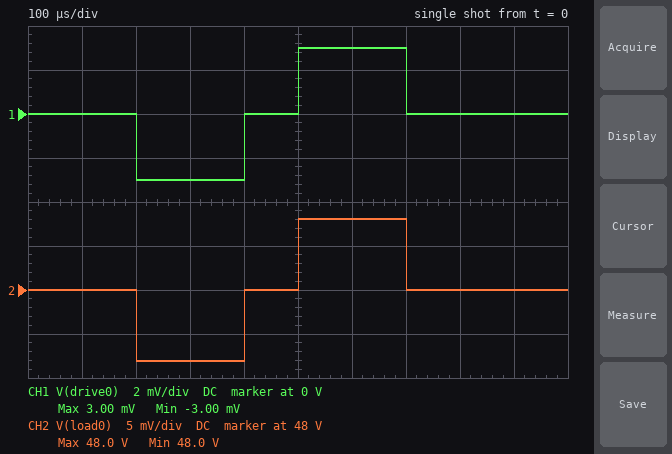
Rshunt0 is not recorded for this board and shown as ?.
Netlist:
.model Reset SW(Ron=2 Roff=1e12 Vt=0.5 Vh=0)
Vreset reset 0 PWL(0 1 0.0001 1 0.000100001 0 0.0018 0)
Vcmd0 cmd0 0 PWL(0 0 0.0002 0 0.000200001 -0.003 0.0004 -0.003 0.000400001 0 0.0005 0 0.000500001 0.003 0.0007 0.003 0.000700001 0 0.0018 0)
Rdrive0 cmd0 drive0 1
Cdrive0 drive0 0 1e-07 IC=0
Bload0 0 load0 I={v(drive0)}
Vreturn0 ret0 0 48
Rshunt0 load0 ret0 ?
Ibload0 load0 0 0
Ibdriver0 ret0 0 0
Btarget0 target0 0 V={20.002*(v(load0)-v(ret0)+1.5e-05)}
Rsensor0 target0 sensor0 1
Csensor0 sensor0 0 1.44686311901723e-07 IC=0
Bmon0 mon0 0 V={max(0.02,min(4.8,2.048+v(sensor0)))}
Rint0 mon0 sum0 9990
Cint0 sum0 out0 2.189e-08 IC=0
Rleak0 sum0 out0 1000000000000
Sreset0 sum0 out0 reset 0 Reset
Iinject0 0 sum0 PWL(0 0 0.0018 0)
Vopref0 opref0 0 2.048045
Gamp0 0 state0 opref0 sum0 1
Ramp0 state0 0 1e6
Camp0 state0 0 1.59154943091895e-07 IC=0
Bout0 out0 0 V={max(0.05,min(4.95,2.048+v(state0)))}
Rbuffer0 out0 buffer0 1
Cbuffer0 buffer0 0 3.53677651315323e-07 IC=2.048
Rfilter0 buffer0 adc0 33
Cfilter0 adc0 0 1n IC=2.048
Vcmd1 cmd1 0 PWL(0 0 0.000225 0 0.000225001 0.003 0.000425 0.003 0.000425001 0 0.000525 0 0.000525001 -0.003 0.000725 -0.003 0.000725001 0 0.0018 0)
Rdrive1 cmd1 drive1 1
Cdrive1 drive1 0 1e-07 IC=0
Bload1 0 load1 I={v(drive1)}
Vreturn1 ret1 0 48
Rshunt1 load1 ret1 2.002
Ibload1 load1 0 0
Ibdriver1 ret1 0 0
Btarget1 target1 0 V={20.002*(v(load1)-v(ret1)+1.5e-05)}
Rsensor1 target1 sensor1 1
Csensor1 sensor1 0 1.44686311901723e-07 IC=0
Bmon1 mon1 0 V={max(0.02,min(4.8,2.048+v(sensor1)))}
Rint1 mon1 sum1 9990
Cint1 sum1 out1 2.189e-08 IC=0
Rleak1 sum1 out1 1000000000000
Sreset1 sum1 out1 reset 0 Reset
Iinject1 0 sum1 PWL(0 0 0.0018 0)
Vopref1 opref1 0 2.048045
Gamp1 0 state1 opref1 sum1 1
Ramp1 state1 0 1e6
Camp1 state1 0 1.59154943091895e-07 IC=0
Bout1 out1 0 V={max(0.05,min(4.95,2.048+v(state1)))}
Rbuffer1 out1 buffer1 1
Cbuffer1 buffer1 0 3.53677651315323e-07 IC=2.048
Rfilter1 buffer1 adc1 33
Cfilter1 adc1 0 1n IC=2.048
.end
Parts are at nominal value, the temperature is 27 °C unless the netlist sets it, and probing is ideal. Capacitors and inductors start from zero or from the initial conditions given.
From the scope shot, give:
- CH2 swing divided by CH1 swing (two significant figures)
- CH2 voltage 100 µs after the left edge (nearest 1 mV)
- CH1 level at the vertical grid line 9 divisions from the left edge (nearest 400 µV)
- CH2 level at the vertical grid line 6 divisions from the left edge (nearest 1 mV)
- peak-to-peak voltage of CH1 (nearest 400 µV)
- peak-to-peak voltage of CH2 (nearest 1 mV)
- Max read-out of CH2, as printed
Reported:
2.7
48.000 V
0 V
48.008 V
6.0 mV
16 mV
48.0 V
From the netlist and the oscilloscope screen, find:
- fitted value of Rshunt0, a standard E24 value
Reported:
2.7 Ω
